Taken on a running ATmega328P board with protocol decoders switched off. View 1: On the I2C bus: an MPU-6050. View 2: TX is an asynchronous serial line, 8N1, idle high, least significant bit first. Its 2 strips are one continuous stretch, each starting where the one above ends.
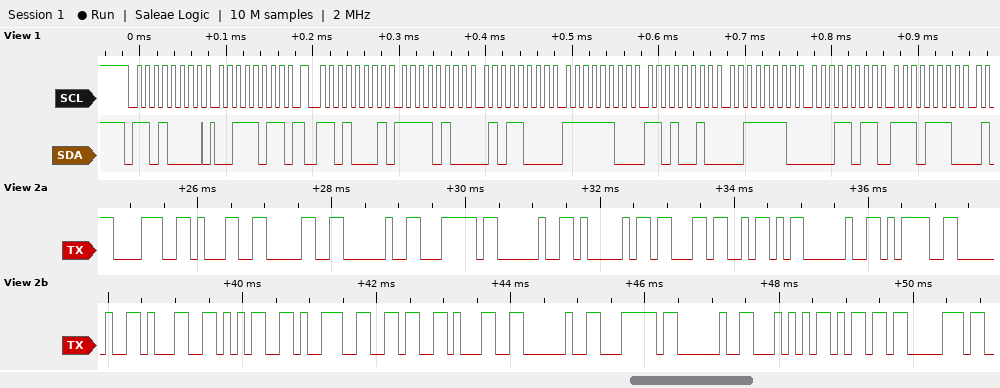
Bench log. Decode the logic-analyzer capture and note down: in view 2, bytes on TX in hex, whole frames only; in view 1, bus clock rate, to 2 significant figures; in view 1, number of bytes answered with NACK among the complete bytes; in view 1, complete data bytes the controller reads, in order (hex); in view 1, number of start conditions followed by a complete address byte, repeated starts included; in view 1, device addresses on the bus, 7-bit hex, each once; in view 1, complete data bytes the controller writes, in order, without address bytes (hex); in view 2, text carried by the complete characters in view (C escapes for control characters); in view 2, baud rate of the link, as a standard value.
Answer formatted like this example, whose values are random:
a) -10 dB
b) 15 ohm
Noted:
a) 38 31 30 20 7C 20 41 63 5A 20 3D 20 31 35 39 36 31 20 7C 20 54 6D 70
b) 100 kHz
c) 0
d) F4 58 FC D2 3E 1B EE
e) 2
f) 0x68
g) 3B
h) "810 | AcZ = 15961 | Tmp"
i) 9600 baud
